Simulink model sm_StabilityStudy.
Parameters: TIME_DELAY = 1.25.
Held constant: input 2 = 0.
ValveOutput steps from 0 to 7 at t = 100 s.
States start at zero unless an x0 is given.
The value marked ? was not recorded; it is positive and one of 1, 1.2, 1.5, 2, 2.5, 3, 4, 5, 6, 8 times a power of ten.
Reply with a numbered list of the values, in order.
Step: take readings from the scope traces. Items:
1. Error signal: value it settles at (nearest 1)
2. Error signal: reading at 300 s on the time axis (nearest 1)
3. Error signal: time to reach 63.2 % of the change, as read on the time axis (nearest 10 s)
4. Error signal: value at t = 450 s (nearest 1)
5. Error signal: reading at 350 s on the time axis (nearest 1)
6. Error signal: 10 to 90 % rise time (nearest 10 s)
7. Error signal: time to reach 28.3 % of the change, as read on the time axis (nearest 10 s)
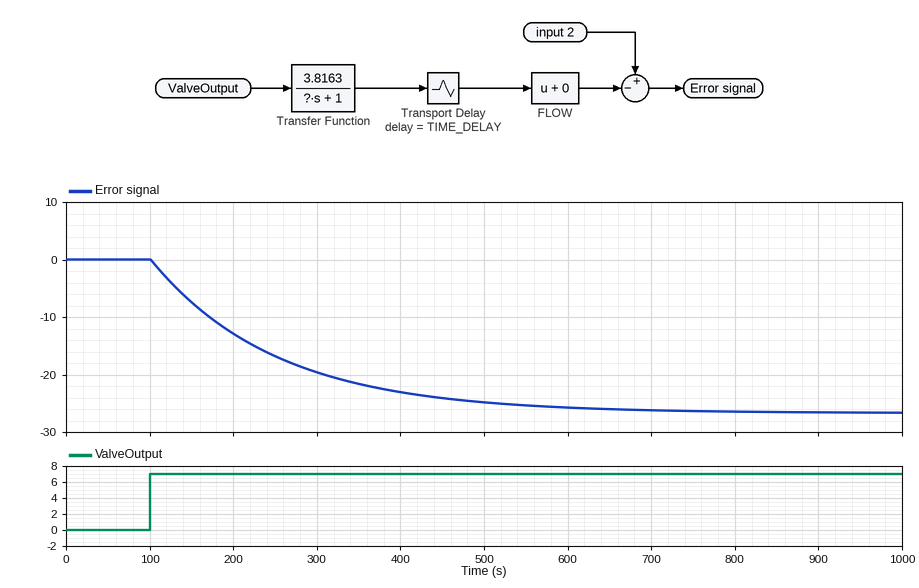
1. -27
2. -20
3. 250 s
4. -24
5. -22
6. 330 s
7. 150 s
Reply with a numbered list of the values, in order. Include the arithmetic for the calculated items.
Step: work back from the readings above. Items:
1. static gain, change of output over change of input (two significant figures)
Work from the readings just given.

1. (-27 - 0) / (7 - 0) = -3.9
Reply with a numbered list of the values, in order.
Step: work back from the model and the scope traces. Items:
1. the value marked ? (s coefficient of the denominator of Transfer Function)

1. 150
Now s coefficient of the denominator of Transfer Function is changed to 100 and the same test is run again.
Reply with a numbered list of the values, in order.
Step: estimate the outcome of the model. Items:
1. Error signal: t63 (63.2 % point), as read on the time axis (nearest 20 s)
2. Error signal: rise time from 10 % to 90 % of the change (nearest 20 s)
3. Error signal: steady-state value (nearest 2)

1. 200 s
2. 220 s
3. -26
